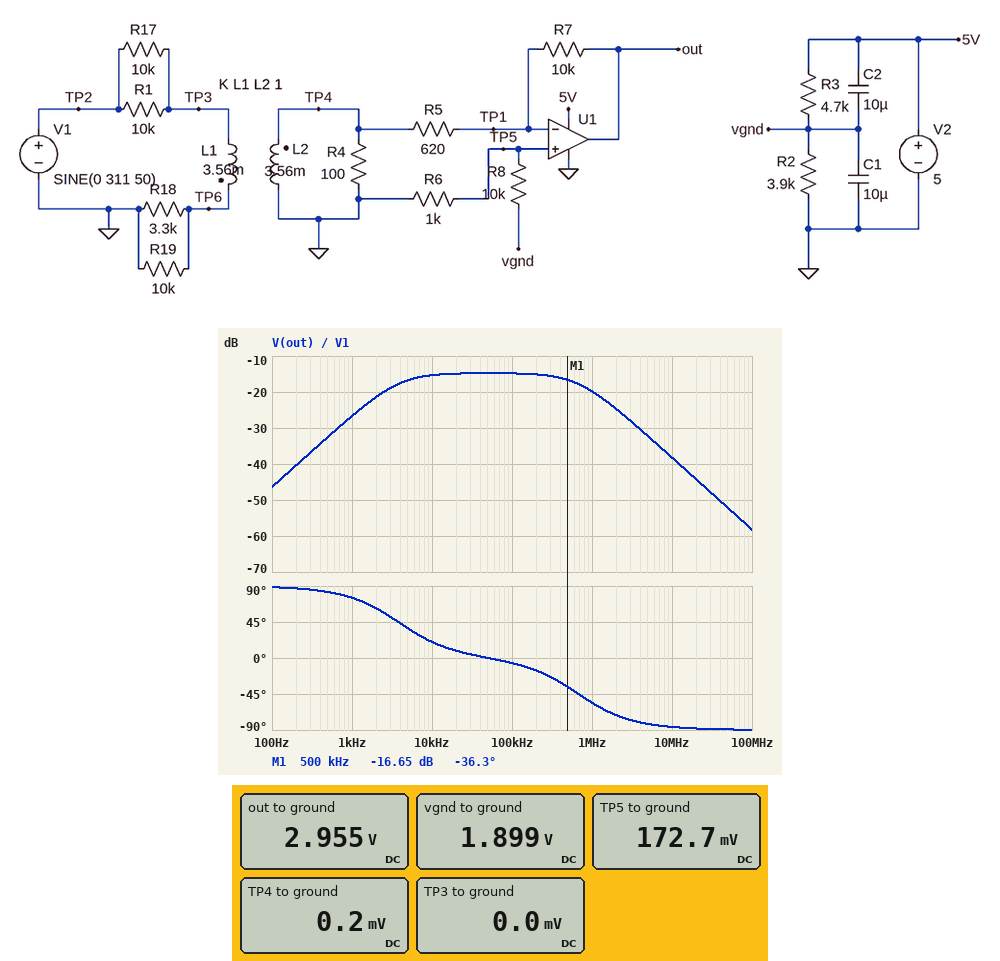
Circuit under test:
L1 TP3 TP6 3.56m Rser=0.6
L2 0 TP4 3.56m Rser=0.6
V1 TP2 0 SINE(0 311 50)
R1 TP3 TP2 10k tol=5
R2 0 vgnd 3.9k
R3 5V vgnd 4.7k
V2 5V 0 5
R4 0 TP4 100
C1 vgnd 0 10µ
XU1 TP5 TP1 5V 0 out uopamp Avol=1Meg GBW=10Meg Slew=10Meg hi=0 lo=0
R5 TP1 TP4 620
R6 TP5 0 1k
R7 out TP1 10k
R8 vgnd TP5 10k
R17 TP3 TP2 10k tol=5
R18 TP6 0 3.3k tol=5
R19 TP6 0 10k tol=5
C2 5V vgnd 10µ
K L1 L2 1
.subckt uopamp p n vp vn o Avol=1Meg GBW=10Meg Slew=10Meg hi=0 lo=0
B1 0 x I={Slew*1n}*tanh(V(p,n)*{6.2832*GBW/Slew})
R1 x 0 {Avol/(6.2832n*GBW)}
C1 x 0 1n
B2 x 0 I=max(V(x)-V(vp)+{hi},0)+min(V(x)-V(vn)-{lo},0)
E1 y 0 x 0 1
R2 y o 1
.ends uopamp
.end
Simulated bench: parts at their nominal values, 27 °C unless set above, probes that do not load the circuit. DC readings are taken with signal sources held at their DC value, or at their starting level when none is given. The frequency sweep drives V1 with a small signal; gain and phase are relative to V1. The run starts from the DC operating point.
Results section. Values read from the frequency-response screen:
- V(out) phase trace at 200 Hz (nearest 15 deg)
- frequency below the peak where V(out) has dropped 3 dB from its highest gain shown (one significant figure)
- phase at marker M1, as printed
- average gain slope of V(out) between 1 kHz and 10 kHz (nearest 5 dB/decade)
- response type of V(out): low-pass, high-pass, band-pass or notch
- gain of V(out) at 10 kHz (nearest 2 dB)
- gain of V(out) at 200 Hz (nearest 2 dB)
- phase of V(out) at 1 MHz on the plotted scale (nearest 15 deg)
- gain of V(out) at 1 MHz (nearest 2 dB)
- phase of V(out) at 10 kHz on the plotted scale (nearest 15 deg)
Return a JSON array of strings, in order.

["90 deg", "4 kHz", "-36.3 deg", "10 dB/decade", "band-pass", "-16 dB", "-40 dB", "-60 deg", "-20 dB", "15 deg"]
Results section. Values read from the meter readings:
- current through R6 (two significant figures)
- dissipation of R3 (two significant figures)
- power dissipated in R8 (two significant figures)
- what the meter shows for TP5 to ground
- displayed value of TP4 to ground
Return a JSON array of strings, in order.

["170 µA", "2.0 mW", "300 µW", "172.7 mV", "0.2 mV"]
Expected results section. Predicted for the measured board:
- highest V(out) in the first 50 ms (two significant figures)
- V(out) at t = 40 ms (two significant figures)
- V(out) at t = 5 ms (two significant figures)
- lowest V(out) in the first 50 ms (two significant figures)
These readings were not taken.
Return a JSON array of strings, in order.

["3.7 V", "3.7 V", "3.0 V", "2.2 V"]
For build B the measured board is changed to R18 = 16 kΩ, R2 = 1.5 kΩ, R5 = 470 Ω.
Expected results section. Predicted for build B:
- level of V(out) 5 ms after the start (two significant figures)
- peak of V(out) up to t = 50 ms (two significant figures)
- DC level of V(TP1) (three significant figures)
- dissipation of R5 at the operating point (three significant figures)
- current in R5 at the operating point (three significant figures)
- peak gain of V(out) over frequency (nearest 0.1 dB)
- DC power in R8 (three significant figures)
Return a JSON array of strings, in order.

["2.2 V", "2.9 V", "99.7 mV", "21.1 µW", "212 µA", "-16.2 dB", "99.3 µW"]
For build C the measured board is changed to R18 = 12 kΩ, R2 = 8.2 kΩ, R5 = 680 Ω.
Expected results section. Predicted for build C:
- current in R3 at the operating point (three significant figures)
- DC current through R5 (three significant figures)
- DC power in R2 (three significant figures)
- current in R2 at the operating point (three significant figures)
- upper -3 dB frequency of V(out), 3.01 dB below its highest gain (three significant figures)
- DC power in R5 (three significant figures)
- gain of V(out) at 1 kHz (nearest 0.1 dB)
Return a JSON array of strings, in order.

["532 µA", "334 µA", "762 µW", "305 µA", "731 kHz", "75.8 µW", "-30.4 dB"]
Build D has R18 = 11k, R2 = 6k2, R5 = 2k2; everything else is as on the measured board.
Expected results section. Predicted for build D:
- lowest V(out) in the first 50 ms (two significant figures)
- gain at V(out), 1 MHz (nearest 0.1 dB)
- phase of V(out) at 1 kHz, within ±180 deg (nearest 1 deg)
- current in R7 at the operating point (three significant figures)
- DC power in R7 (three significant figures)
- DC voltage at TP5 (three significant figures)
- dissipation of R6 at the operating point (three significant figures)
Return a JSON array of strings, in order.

["1.0 V", "-28.6 dB", "77 deg", "94.5 µA", "89.3 µW", "208 mV", "43.3 µW"]
